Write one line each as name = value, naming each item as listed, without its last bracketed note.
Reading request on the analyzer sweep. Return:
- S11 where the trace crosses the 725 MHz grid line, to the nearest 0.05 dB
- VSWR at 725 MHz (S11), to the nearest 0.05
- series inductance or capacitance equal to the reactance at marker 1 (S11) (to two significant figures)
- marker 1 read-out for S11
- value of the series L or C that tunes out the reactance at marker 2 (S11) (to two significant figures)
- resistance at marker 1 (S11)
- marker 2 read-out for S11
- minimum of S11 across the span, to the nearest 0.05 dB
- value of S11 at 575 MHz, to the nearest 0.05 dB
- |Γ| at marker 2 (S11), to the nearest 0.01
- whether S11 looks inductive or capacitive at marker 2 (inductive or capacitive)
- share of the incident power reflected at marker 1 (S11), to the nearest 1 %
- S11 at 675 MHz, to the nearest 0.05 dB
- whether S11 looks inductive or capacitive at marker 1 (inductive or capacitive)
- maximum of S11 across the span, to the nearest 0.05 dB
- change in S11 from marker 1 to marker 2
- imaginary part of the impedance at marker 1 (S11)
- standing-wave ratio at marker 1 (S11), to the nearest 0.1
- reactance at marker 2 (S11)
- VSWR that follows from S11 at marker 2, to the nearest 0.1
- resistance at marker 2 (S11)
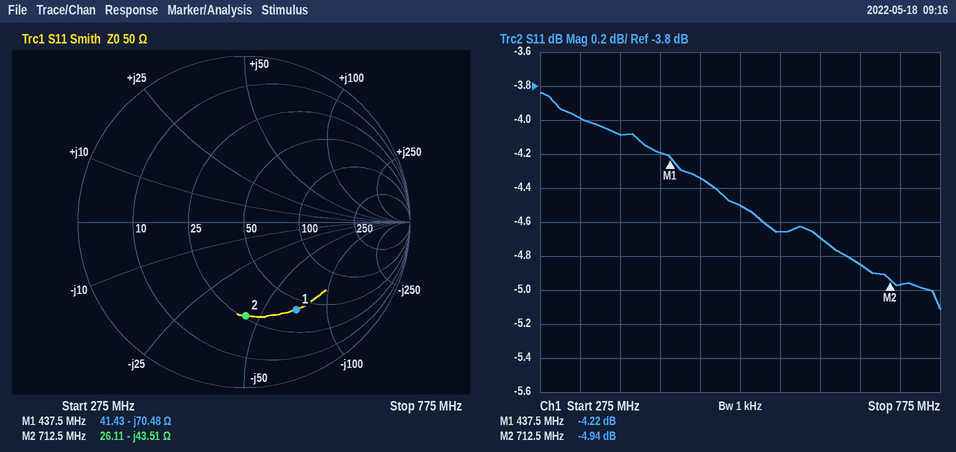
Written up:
S11 where the trace crosses the 725 MHz grid line, to the nearest 0.05 dB = -4.95 dB
VSWR at 725 MHz (S11), to the nearest 0.05 = 3.60
series inductance or capacitance equal to the reactance at marker 1 (S11) = 5.2 pF
marker 1 read-out for S11 = -4.22 dB
value of the series L or C that tunes out the reactance at marker 2 (S11) = 9.7 nH
resistance at marker 1 = 41.43 Ω
marker 2 read-out for S11 = -4.94 dB
minimum of S11 across the span, to the nearest 0.05 dB = -5.10 dB
value of S11 at 575 MHz, to the nearest 0.05 dB = -4.65 dB
|Γ| at marker 2 (S11), to the nearest 0.01 = 0.57
whether S11 looks inductive or capacitive at marker 2 = capacitive
share of the incident power reflected at marker 1 (S11), to the nearest 1 % = 38 %
S11 at 675 MHz, to the nearest 0.05 dB = -4.85 dB
whether S11 looks inductive or capacitive at marker 1 = capacitive
maximum of S11 across the span, to the nearest 0.05 dB = -3.85 dB
change in S11 from marker 1 to marker 2 = -0.72 dB
imaginary part of the impedance at marker 1 = -70.48 Ω
standing-wave ratio at marker 1 (S11), to the nearest 0.1 = 4.2
reactance at marker 2 = -43.51 Ω
VSWR that follows from S11 at marker 2, to the nearest 0.1 = 3.6
resistance at marker 2 = 26.11 Ω
